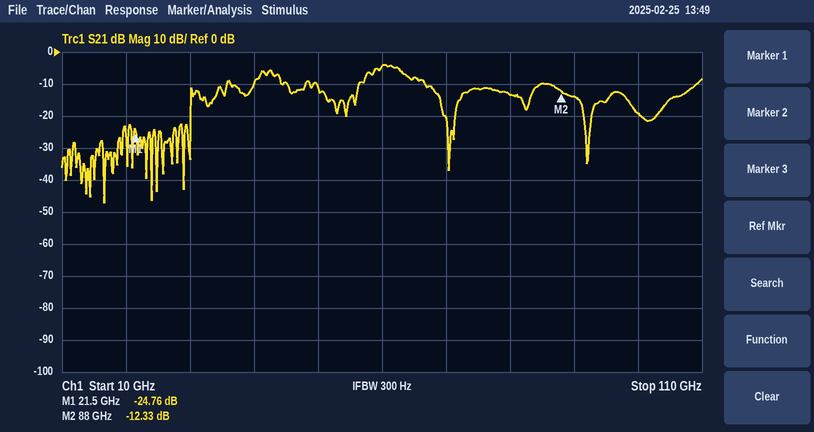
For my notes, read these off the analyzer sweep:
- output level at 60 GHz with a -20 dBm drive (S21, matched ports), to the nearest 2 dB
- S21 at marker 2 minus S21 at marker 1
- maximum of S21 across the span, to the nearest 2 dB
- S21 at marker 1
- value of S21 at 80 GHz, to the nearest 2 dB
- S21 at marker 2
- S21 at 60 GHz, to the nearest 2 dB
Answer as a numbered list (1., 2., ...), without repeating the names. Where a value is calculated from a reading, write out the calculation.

1. -20 dBm + (-4 dB) = -24 dBm
2. -12.33 − (-24.76) = 12.43 dB
3. -4 dB
4. -24.76 dB
5. -14 dB
6. -12.33 dB
7. -4 dB
